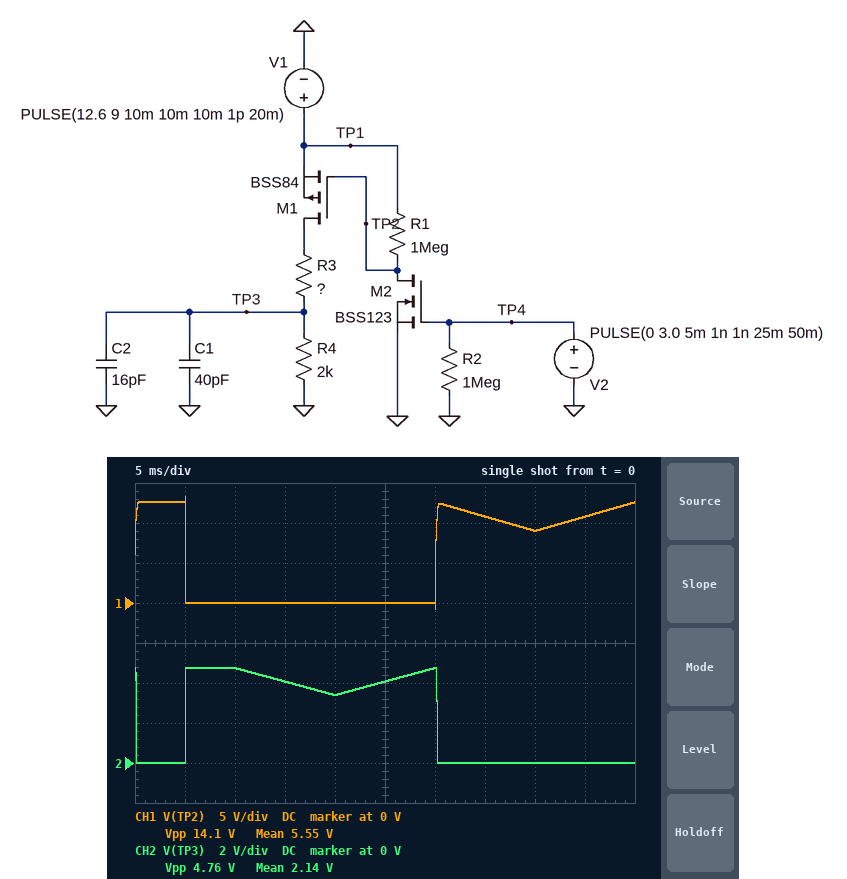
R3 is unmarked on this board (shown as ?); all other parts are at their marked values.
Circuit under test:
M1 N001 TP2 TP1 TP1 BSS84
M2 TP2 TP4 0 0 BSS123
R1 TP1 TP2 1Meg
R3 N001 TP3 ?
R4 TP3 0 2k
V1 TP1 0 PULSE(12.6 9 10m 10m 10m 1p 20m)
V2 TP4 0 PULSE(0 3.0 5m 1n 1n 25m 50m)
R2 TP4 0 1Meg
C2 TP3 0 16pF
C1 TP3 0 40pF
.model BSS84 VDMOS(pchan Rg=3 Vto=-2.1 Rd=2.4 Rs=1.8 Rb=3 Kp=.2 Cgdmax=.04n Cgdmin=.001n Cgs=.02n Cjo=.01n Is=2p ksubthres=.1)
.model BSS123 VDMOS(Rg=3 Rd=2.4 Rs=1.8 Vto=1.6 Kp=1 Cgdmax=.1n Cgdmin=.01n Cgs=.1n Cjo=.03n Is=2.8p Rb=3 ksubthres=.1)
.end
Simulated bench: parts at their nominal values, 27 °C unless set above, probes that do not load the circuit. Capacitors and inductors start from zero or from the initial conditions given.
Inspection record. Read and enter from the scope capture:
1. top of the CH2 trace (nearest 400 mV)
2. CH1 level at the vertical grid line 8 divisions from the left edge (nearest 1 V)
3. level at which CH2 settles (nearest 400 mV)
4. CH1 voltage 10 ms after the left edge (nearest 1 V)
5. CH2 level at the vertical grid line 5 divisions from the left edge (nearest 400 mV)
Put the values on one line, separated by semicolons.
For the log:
4.8 V; 9 V; 0 V; 0 V; 4.0 V
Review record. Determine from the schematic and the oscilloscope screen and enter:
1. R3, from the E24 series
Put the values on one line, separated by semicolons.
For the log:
3.3 kΩ
